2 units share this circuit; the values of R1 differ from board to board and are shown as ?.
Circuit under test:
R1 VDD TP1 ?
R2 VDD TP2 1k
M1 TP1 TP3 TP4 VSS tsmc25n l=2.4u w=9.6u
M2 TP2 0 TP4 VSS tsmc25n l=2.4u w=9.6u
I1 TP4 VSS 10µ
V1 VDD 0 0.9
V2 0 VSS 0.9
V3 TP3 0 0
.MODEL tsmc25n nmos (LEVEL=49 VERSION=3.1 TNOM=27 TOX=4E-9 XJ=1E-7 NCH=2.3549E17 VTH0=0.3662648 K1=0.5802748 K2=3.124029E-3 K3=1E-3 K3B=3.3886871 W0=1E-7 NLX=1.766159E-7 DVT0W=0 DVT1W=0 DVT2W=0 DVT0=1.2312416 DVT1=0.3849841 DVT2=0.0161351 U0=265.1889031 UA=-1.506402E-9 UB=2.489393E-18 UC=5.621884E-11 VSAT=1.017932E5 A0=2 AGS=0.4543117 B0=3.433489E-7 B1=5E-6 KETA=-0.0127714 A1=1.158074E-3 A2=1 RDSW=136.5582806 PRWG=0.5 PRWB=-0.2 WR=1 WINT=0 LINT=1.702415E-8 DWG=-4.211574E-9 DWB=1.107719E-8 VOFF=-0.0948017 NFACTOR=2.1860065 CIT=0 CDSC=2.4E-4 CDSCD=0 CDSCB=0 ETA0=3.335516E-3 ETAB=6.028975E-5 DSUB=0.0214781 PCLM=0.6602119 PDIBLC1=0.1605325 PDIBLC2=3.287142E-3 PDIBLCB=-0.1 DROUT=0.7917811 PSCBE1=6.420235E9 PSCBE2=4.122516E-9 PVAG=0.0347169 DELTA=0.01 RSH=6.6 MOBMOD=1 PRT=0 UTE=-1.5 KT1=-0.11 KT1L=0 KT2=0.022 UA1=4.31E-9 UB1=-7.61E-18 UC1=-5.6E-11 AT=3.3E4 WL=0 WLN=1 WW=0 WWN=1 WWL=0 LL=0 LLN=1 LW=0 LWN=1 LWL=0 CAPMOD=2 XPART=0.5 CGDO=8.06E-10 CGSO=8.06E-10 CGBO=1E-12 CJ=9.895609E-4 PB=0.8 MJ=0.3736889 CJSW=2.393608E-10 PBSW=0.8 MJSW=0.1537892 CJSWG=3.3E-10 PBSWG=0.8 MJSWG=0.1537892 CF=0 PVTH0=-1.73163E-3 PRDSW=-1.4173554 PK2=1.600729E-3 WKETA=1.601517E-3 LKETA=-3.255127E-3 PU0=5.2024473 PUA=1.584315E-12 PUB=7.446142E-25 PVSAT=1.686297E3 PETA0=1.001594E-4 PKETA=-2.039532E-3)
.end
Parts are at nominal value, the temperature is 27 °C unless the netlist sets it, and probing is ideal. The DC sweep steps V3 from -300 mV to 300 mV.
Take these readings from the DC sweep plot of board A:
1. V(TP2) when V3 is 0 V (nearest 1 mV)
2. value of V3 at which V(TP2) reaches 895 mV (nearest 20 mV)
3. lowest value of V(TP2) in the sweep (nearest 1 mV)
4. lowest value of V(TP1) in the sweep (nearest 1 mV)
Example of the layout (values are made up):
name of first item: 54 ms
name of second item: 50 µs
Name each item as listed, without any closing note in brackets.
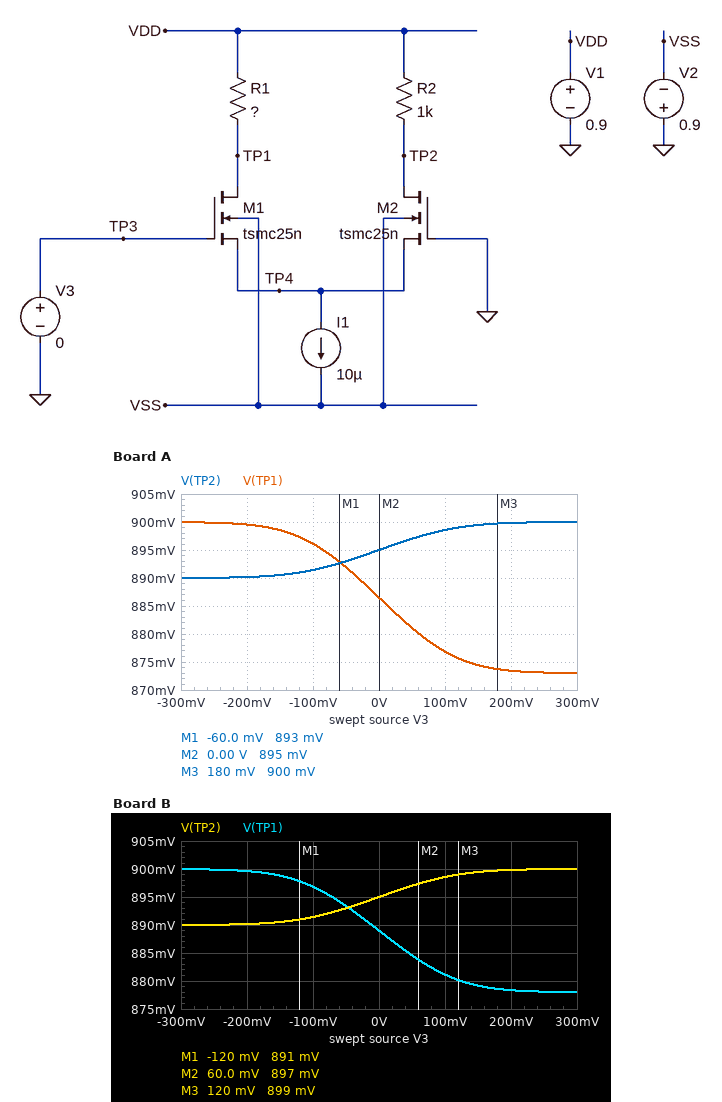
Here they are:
V(TP2) when V3 is 0 V: 895 mV
value of V3 at which V(TP2) reaches 895 mV: 0 V
lowest value of V(TP2) in the sweep: 890 mV
lowest value of V(TP1) in the sweep: 873 mV
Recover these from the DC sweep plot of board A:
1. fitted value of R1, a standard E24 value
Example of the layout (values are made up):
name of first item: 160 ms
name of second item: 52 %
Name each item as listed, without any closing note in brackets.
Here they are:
fitted value of R1, a standard E24 value: 2.7 kΩ
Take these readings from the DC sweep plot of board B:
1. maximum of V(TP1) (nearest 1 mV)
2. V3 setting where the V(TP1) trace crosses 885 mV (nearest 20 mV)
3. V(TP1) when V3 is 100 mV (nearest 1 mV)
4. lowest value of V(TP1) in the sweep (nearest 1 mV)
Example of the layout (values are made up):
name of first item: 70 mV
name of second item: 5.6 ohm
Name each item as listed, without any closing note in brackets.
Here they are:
maximum of V(TP1): 900 mV
V3 setting where the V(TP1) trace crosses 885 mV: 40 mV
V(TP1) when V3 is 100 mV: 881 mV
lowest value of V(TP1) in the sweep: 878 mV
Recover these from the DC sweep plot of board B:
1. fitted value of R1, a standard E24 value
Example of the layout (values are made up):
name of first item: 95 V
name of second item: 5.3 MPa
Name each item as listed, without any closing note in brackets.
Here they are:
fitted value of R1, a standard E24 value: 2.2 kΩ
